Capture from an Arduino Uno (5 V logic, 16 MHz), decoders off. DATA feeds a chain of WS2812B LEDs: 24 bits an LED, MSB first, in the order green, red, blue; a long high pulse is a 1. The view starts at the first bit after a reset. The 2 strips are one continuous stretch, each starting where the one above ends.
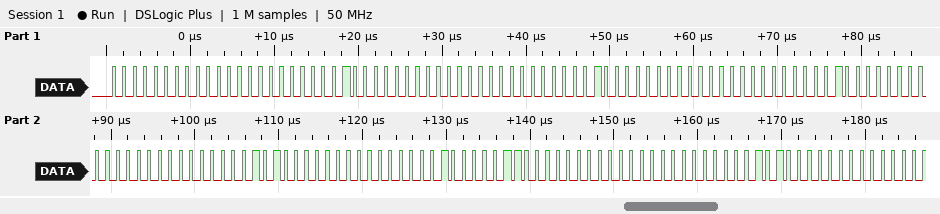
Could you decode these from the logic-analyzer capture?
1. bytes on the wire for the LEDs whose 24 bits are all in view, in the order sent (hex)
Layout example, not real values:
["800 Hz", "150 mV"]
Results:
["00 00 02 00 00 02 00 00 04 00 00 05 00 01 06 00 00 05"]
